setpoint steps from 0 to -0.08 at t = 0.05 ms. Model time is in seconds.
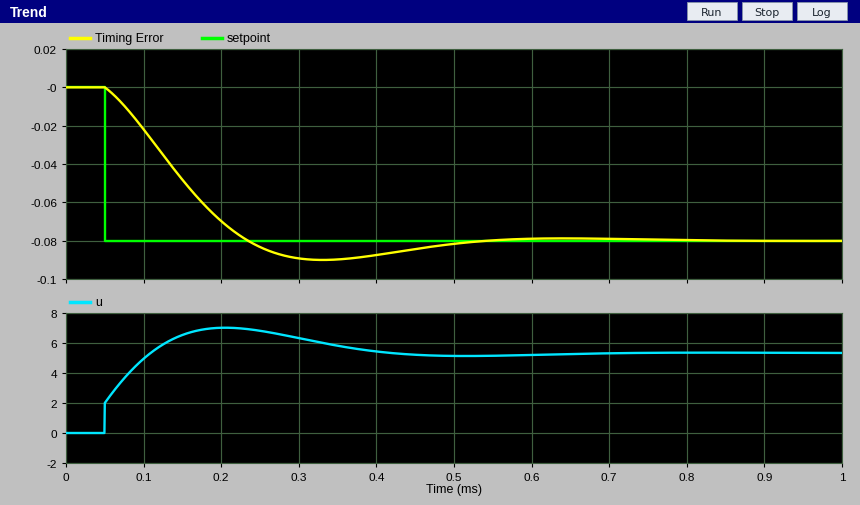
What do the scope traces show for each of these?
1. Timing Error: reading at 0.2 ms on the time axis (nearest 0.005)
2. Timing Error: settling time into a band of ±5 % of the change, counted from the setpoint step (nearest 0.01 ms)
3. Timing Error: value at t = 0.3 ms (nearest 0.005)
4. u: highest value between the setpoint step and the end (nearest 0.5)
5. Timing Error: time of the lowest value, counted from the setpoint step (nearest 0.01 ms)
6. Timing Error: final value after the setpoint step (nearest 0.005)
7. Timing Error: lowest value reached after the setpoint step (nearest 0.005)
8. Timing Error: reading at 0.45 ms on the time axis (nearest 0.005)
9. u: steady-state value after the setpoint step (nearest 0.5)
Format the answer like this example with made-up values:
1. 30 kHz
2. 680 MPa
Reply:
1. -0.070
2. 0.41 ms
3. -0.090
4. 7.0
5. 0.28 ms
6. -0.080
7. -0.090
8. -0.085
9. 5.5
